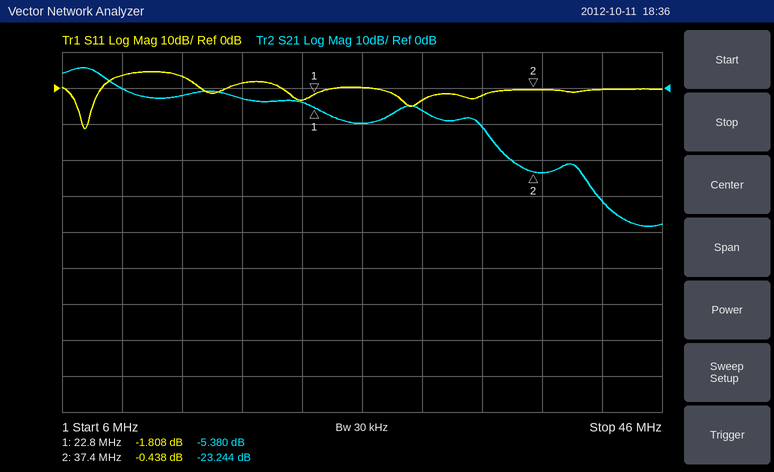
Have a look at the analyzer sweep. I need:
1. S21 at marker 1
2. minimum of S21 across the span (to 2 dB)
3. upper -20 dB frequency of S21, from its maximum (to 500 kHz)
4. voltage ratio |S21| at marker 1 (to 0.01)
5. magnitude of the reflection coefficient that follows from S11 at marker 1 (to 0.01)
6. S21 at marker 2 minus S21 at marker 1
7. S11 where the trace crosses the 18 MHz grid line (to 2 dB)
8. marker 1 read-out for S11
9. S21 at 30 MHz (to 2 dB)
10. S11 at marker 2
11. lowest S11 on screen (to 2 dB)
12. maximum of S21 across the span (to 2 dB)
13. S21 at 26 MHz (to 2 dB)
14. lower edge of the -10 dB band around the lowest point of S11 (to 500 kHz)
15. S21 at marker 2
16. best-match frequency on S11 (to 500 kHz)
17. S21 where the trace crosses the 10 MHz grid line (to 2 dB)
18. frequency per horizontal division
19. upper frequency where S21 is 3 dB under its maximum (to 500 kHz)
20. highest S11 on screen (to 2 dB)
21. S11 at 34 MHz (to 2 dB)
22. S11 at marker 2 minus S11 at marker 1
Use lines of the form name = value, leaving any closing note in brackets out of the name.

S21 at marker 1 = -5.380 dB
minimum of S21 across the span = -38 dB
upper -20 dB frequency of S21, from its maximum = 34.5 MHz
voltage ratio |S21| at marker 1 = 0.54
magnitude of the reflection coefficient that follows from S11 at marker 1 = 0.81
S21 at marker 2 minus S21 at marker 1 = -17.864 dB
S11 where the trace crosses the 18 MHz grid line = 2 dB
marker 1 read-out for S11 = -1.808 dB
S21 at 30 MHz = -6 dB
S11 at marker 2 = -0.438 dB
lowest S11 on screen = -12 dB
maximum of S21 across the span = 6 dB
S21 at 26 MHz = -10 dB
lower edge of the -10 dB band around the lowest point of S11 = 7.5 MHz
S21 at marker 2 = -23.244 dB
best-match frequency on S11 = 7.5 MHz
S21 where the trace crosses the 10 MHz grid line = 0 dB
frequency per horizontal division = 4 MHz
upper frequency where S21 is 3 dB under its maximum = 9.0 MHz
highest S11 on screen = 4 dB
S11 at 34 MHz = -2 dB
S11 at marker 2 minus S11 at marker 1 = 1.370 dB
